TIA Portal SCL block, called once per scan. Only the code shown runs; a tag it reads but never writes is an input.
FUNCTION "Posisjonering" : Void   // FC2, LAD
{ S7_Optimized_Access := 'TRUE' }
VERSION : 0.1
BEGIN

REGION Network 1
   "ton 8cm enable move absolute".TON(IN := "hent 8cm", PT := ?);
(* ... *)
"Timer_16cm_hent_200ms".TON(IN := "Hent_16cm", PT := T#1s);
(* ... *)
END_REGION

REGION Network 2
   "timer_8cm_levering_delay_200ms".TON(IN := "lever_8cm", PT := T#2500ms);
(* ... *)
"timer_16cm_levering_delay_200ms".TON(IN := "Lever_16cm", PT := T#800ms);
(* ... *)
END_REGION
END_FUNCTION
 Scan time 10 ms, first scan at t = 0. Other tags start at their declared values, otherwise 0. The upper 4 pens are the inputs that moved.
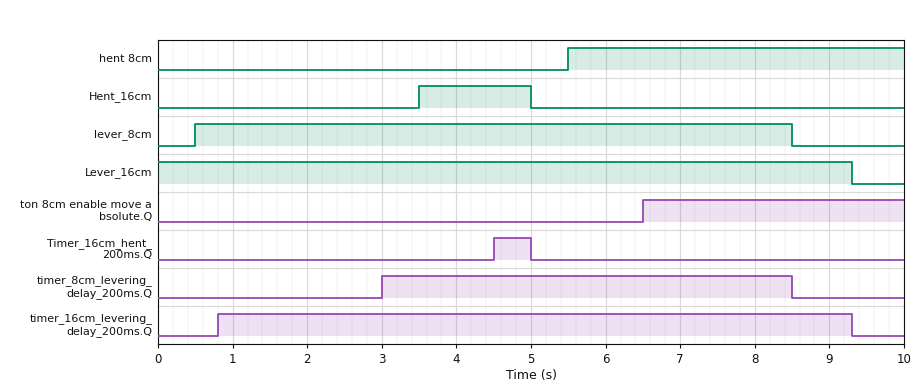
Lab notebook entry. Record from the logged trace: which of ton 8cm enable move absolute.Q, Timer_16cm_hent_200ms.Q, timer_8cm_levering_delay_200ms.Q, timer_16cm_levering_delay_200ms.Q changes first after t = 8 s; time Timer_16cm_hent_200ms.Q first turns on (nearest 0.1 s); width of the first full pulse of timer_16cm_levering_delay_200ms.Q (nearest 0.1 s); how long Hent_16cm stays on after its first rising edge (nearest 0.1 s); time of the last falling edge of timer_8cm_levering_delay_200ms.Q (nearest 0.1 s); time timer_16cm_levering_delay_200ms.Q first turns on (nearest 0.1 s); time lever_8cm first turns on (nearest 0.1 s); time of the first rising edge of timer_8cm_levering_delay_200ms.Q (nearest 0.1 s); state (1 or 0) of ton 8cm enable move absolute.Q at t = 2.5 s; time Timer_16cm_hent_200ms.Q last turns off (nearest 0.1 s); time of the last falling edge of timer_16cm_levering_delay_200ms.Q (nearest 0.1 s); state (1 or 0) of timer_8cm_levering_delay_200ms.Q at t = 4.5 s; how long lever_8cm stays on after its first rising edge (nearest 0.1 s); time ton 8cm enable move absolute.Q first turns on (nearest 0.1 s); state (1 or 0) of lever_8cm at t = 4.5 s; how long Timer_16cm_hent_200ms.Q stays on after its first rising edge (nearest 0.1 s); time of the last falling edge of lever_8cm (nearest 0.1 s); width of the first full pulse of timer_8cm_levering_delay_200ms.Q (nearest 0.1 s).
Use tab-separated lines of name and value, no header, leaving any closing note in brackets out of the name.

which of ton 8cm enable move absolute.Q, Timer_16cm_hent_200ms.Q, timer_8cm_levering_delay_200ms.Q, timer_16cm_levering_delay_200ms.Q changes first after t = 8 s	timer_8cm_levering_delay_200ms.Q
time Timer_16cm_hent_200ms.Q first turns on	4.5 s
width of the first full pulse of timer_16cm_levering_delay_200ms.Q	8.5 s
how long Hent_16cm stays on after its first rising edge	1.5 s
time of the last falling edge of timer_8cm_levering_delay_200ms.Q	8.5 s
time timer_16cm_levering_delay_200ms.Q first turns on	0.8 s
time lever_8cm first turns on	0.5 s
time of the first rising edge of timer_8cm_levering_delay_200ms.Q	3.0 s
state (1 or 0) of ton 8cm enable move absolute.Q at t = 2.5 s	0
time Timer_16cm_hent_200ms.Q last turns off	5.0 s
time of the last falling edge of timer_16cm_levering_delay_200ms.Q	9.3 s
state (1 or 0) of timer_8cm_levering_delay_200ms.Q at t = 4.5 s	1
how long lever_8cm stays on after its first rising edge	8.0 s
time ton 8cm enable move absolute.Q first turns on	6.5 s
state (1 or 0) of lever_8cm at t = 4.5 s	1
how long Timer_16cm_hent_200ms.Q stays on after its first rising edge	0.5 s
time of the last falling edge of lever_8cm	8.5 s
width of the first full pulse of timer_8cm_levering_delay_200ms.Q	5.5 s
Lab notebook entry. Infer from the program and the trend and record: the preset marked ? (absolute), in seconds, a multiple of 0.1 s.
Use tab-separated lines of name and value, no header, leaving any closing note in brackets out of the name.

the preset marked ? (absolute), in seconds, a multiple of 0.1 s	1.0 s
